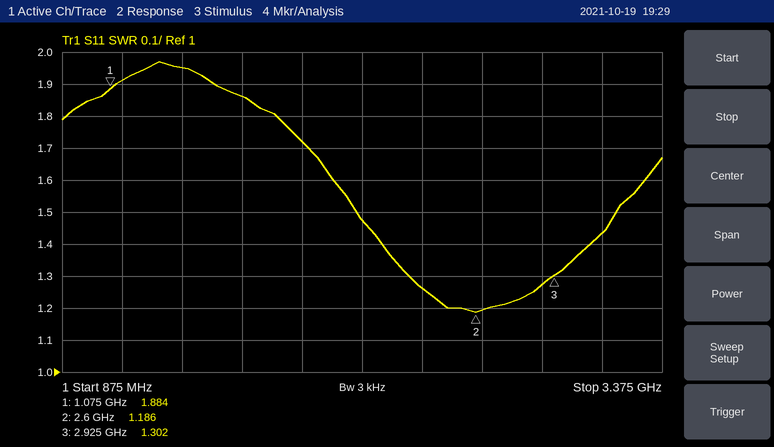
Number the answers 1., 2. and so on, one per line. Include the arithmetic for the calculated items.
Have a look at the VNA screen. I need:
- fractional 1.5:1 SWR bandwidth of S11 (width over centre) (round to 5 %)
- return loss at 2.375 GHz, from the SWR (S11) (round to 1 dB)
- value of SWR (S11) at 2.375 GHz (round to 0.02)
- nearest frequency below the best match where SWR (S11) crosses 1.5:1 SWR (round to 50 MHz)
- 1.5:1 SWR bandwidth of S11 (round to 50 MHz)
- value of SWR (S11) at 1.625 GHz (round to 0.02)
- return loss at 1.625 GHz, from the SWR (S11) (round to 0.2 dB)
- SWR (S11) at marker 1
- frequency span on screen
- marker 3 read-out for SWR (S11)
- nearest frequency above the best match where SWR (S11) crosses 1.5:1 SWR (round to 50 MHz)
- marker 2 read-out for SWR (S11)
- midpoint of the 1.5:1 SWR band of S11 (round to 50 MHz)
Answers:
1. 1.1 GHz / 2.65 GHz ≈ 41.5 %, so 40 % to the nearest 5 %
2. −20 log10((1.26 − 1)/(1.26 + 1)) ≈ 19 dB
3. 1.26
4. 2.10 GHz
5. 3.20 GHz − 2.10 GHz = 1.10 GHz
6. 1.86
7. −20 log10((1.86 − 1)/(1.86 + 1)) ≈ 10.4 dB
8. 1.884
9. 2.5 GHz
10. 1.302
11. 3.20 GHz
12. 1.186
13. 2.65 GHz
